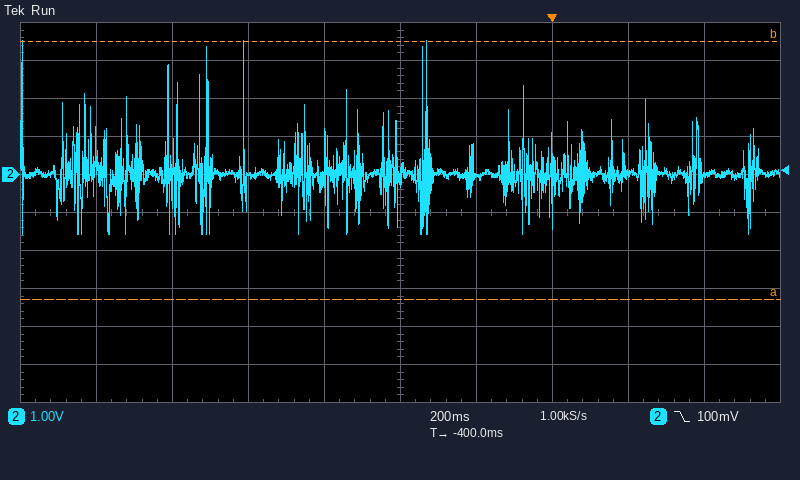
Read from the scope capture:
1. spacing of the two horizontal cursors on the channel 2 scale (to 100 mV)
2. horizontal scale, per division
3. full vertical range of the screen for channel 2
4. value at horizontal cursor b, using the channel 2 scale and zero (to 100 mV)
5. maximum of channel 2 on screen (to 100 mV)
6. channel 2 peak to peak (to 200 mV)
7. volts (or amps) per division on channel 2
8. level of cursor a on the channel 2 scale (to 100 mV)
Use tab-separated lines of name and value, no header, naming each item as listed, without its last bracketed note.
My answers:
spacing of the two horizontal cursors on the channel 2 scale	6.8 V
horizontal scale, per division	200 ms
full vertical range of the screen for channel 2	10 V
value at horizontal cursor b, using the channel 2 scale and zero	3.5 V
maximum of channel 2 on screen	3.5 V
channel 2 peak to peak	5.0 V
volts (or amps) per division on channel 2	1 V
level of cursor a on the channel 2 scale	-3.3 V
